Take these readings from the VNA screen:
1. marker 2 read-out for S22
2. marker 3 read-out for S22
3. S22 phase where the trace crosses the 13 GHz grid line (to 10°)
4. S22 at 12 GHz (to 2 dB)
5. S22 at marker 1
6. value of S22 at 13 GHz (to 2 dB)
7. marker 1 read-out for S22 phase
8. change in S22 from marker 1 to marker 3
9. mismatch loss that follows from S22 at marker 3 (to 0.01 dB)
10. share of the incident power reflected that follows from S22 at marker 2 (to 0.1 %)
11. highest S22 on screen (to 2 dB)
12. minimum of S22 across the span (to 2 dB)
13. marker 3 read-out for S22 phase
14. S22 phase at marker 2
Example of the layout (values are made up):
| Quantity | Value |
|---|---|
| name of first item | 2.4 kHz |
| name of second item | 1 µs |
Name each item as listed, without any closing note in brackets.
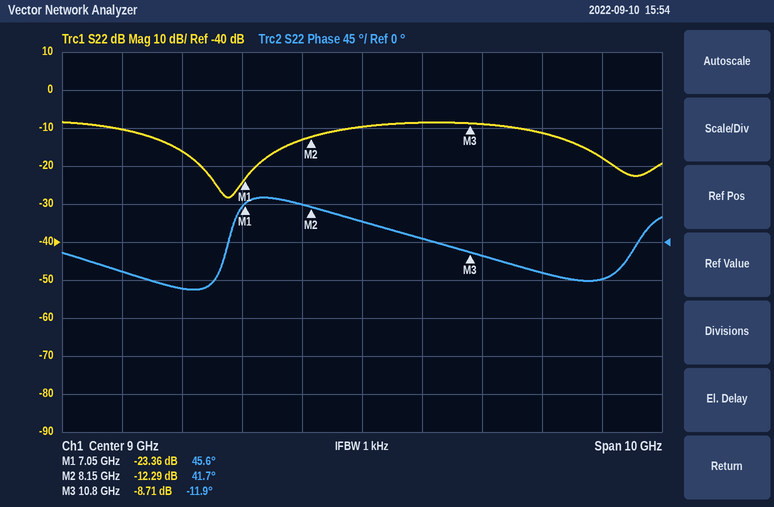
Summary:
| Quantity | Value |
|---|---|
| marker 2 read-out for S22 | -12.29 dB |
| marker 3 read-out for S22 | -8.71 dB |
| S22 phase where the trace crosses the 13 GHz grid line | -40° |
| S22 at 12 GHz | -12 dB |
| S22 at marker 1 | -23.36 dB |
| value of S22 at 13 GHz | -18 dB |
| marker 1 read-out for S22 phase | 45.6° |
| change in S22 from marker 1 to marker 3 | 14.65 dB |
| mismatch loss that follows from S22 at marker 3 | 0.63 dB |
| share of the incident power reflected that follows from S22 at marker 2 | 5.9 % |
| highest S22 on screen | -8 dB |
| minimum of S22 across the span | -28 dB |
| marker 3 read-out for S22 phase | -11.9° |
| S22 phase at marker 2 | 41.7° |
